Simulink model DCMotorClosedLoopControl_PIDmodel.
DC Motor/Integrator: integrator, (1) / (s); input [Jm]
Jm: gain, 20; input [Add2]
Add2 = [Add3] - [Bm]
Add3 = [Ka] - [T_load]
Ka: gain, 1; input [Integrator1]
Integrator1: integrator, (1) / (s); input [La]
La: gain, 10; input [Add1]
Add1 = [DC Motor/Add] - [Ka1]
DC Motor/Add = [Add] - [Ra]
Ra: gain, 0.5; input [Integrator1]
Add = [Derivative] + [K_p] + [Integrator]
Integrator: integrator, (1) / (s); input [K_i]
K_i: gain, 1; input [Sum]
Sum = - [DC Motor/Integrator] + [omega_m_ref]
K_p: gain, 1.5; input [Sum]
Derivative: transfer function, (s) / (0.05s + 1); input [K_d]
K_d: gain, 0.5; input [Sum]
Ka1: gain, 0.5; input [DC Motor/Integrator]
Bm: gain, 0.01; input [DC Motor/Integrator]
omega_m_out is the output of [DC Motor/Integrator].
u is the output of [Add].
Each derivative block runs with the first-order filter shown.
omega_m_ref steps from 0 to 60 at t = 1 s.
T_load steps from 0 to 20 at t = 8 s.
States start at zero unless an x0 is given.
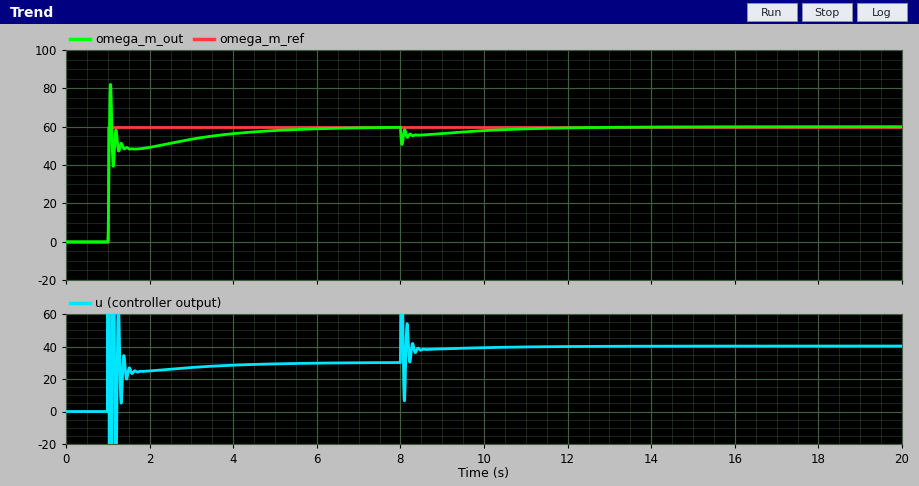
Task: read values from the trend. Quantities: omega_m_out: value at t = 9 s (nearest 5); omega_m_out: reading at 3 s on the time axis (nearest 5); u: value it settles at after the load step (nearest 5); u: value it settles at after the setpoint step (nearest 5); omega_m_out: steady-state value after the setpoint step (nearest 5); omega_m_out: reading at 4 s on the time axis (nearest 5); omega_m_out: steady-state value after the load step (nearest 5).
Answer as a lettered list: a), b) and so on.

a) 55
b) 55
c) 40
d) 30
e) 60
f) 55
g) 60
